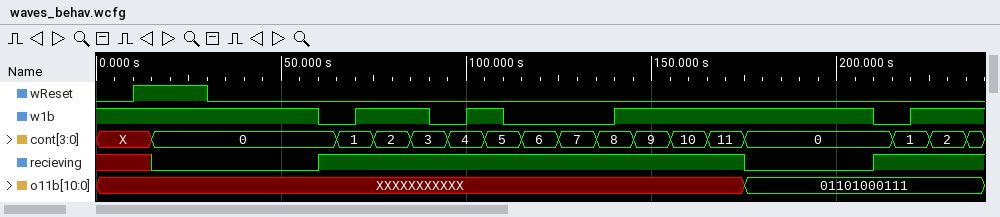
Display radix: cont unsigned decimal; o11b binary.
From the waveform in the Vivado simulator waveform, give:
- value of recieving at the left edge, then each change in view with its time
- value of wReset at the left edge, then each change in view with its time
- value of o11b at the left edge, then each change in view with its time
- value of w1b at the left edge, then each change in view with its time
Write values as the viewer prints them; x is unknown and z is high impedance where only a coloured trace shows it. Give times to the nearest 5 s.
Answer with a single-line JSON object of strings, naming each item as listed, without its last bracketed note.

{"value of recieving at the left edge, then each change in view with its time": "x, 0 at 15 s, 1 at 60 s, 0 at 175 s, 1 at 210 s", "value of wReset at the left edge, then each change in view with its time": "0, 1 at 10 s, 0 at 30 s", "value of o11b at the left edge, then each change in view with its time": "XXXXXXXXXXX, 01101000111 at 175 s", "value of w1b at the left edge, then each change in view with its time": "1, 0 at 60 s, 1 at 70 s, 0 at 90 s, 1 at 100 s, 0 at 110 s, 1 at 140 s, 0 at 210 s, 1 at 220 s"}
